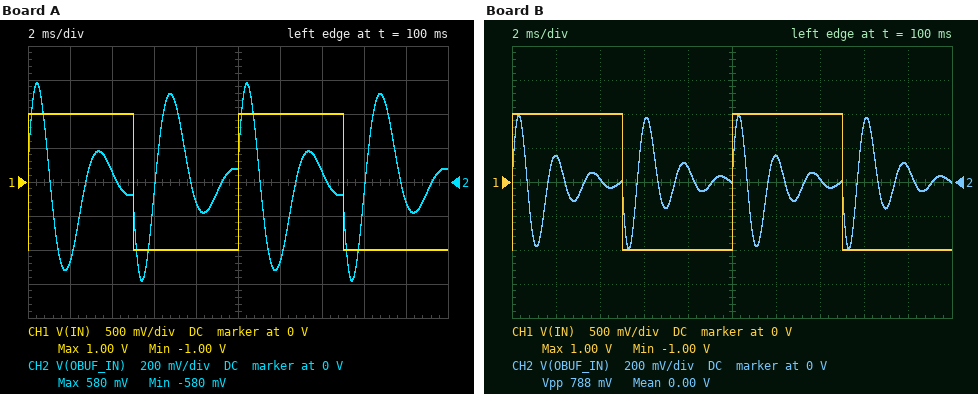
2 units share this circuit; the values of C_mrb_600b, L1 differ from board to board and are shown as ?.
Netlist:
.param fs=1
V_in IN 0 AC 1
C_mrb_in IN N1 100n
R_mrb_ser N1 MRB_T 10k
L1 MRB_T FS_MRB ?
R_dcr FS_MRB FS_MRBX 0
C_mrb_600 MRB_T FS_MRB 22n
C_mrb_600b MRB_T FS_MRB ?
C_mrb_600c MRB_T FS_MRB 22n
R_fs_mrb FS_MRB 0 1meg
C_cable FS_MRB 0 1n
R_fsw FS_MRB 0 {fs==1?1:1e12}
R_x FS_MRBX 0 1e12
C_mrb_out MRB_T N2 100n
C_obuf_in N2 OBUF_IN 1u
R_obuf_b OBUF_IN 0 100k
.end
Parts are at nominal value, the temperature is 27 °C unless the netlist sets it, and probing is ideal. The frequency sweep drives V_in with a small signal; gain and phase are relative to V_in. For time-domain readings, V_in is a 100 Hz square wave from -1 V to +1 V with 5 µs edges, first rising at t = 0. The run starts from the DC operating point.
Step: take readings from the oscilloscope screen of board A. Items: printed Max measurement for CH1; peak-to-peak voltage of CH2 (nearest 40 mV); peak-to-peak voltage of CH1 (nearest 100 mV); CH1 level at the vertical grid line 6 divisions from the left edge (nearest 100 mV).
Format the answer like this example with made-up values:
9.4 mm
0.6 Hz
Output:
1.00 V
1.16 V
2.0 V
1.0 V
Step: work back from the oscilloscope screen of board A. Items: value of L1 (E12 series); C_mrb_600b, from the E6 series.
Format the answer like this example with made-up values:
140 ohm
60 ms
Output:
2.2 H
33 nF
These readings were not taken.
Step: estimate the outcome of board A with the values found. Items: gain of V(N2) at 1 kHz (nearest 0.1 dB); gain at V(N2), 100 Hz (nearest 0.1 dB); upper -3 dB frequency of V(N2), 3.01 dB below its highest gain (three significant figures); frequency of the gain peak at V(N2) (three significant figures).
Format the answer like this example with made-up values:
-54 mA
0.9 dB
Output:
-13.0 dB
-21.6 dB
456 Hz
346 Hz
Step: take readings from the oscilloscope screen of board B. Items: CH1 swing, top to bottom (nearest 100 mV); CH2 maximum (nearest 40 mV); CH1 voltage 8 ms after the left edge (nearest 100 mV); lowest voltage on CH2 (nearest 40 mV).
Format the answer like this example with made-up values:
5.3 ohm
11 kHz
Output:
2.0 V
400 mV
-1.0 V
-400 mV
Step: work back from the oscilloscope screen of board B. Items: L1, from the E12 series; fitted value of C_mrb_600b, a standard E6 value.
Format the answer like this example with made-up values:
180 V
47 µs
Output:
820 mH
33 nF
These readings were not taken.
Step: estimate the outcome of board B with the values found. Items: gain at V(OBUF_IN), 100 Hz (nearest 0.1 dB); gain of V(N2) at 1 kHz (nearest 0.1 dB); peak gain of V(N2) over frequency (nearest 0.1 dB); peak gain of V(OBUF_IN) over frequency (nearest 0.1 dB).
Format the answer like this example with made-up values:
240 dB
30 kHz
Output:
-30.9 dB
-10.3 dB
-0.6 dB
-0.6 dB
